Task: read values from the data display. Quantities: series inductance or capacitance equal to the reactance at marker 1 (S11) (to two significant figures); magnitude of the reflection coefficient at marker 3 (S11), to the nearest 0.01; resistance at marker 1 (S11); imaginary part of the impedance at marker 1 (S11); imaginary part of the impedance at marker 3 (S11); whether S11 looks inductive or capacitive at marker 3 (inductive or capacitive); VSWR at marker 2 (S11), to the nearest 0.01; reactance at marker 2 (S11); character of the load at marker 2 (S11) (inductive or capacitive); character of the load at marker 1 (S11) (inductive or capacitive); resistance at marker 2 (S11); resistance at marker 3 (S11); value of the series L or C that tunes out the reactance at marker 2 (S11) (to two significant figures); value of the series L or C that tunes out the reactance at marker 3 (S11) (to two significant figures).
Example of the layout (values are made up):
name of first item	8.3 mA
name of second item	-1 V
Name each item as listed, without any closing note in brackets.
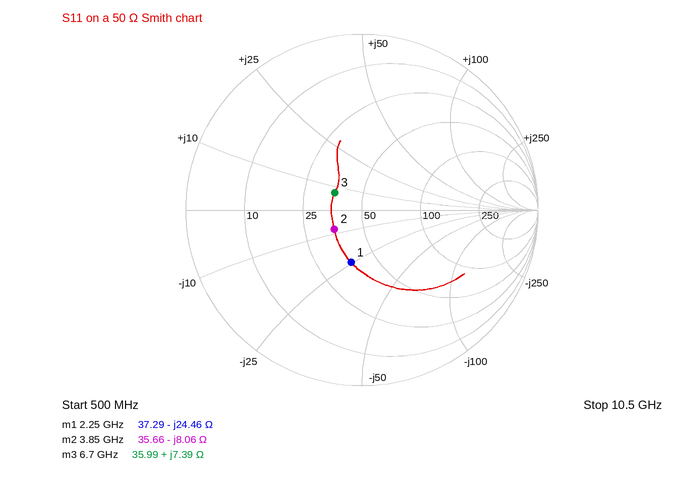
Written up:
series inductance or capacitance equal to the reactance at marker 1 (S11)	2.9 pF
magnitude of the reflection coefficient at marker 3 (S11), to the nearest 0.01	0.18
resistance at marker 1	37.29 Ω
imaginary part of the impedance at marker 1	-24.46 Ω
imaginary part of the impedance at marker 3	+7.39 Ω
whether S11 looks inductive or capacitive at marker 3	inductive
VSWR at marker 2 (S11), to the nearest 0.01	1.47
reactance at marker 2	-8.06 Ω
character of the load at marker 2 (S11)	capacitive
character of the load at marker 1 (S11)	capacitive
resistance at marker 2	35.66 Ω
resistance at marker 3	35.99 Ω
value of the series L or C that tunes out the reactance at marker 2 (S11)	330 pH
value of the series L or C that tunes out the reactance at marker 3 (S11)	3.2 pF
